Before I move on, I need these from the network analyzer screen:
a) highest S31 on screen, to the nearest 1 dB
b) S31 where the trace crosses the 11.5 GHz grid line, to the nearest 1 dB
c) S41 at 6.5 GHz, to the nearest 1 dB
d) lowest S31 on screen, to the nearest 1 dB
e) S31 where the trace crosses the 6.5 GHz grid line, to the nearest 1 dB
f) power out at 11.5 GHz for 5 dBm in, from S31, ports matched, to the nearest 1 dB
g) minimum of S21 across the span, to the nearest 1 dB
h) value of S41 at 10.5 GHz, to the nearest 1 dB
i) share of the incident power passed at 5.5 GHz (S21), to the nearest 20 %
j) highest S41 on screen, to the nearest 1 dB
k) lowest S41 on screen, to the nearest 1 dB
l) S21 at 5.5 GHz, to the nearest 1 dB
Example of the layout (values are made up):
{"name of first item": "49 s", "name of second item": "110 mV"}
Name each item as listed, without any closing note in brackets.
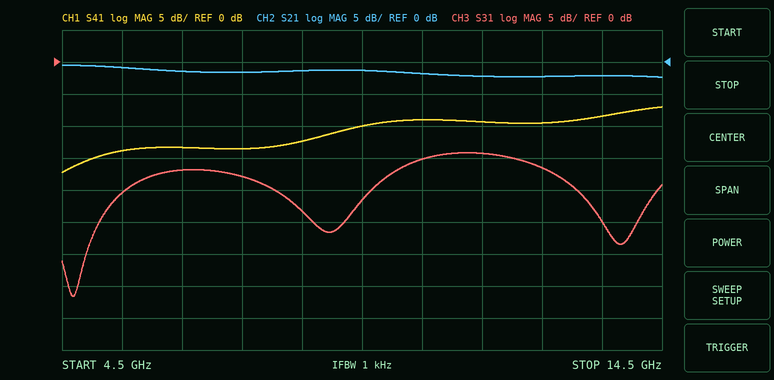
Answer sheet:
{"highest S31 on screen, to the nearest 1 dB": "-14 dB", "S31 where the trace crosses the 11.5 GHz grid line, to the nearest 1 dB": "-14 dB", "S41 at 6.5 GHz, to the nearest 1 dB": "-13 dB", "lowest S31 on screen, to the nearest 1 dB": "-37 dB", "S31 where the trace crosses the 6.5 GHz grid line, to the nearest 1 dB": "-17 dB", "power out at 11.5 GHz for 5 dBm in, from S31, ports matched, to the nearest 1 dB": "-9 dBm", "minimum of S21 across the span, to the nearest 1 dB": "-2 dB", "value of S41 at 10.5 GHz, to the nearest 1 dB": "-9 dB", "share of the incident power passed at 5.5 GHz (S21), to the nearest 20 %": "80 %", "highest S41 on screen, to the nearest 1 dB": "-7 dB", "lowest S41 on screen, to the nearest 1 dB": "-17 dB", "S21 at 5.5 GHz, to the nearest 1 dB": "-1 dB"}
